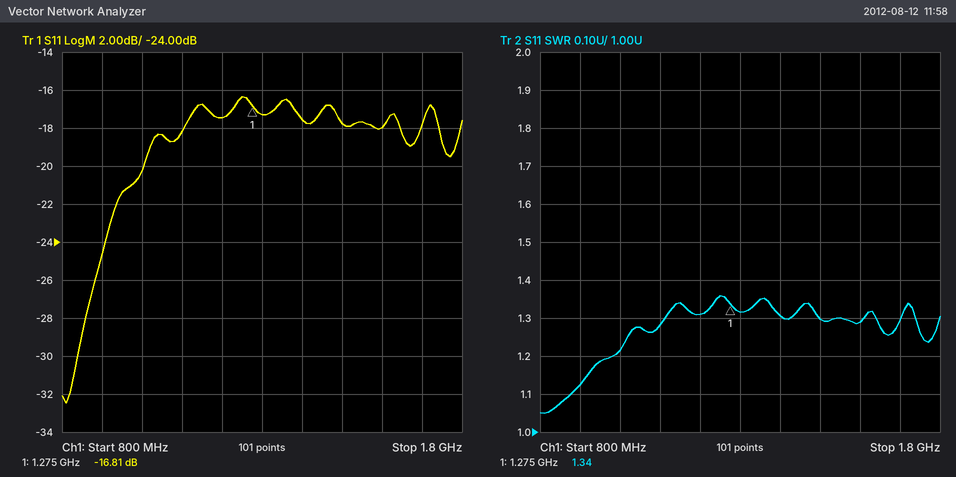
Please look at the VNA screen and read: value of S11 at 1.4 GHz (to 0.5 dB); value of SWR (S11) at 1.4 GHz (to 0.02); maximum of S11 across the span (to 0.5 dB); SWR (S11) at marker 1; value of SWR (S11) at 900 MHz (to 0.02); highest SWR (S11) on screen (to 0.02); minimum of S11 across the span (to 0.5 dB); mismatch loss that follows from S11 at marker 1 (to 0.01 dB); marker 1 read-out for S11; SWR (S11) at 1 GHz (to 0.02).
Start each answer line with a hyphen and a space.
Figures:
- -17.5 dB
- 1.30
- -16.5 dB
- 1.34
- 1.12
- 1.36
- -32.5 dB
- 0.09 dB
- -16.81 dB
- 1.22
